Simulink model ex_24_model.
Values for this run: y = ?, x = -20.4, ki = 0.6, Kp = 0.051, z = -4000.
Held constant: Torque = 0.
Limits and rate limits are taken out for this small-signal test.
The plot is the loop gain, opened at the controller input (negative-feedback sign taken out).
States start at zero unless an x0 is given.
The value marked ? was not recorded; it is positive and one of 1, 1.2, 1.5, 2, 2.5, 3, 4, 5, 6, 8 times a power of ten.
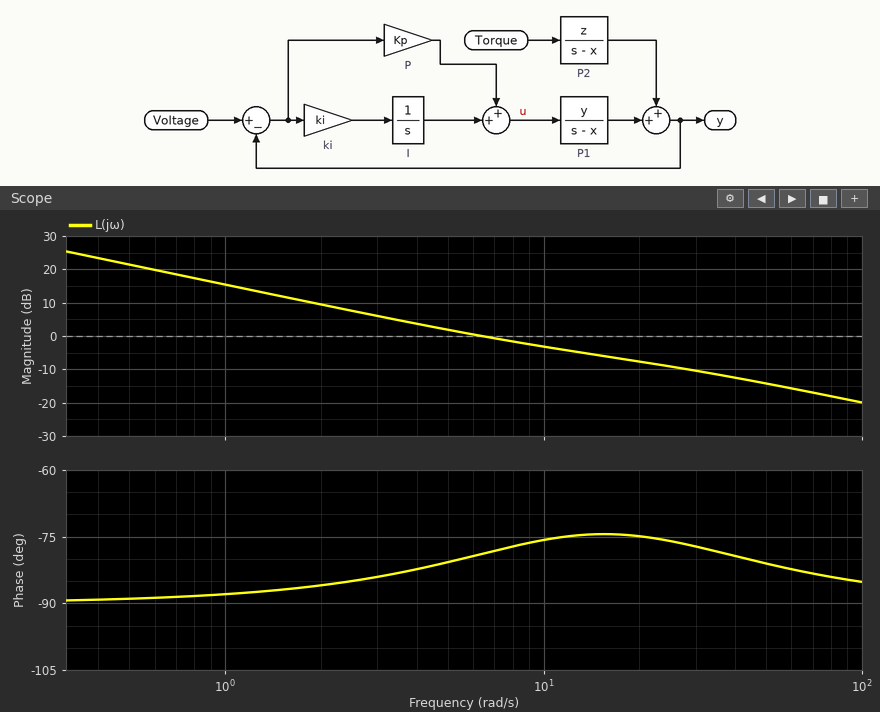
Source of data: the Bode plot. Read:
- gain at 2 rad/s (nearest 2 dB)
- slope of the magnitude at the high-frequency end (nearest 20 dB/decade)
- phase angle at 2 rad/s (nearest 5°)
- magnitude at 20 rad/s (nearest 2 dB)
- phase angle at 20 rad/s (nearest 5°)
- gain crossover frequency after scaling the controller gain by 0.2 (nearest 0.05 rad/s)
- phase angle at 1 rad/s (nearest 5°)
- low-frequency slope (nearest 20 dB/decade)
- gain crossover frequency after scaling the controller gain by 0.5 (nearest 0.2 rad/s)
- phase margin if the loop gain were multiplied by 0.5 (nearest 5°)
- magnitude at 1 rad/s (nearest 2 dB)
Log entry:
10 dB
-20 dB/decade
-85°
-8 dB
-75°
1.20 rad/s
-90°
-20 dB/decade
3.0 rad/s
95°
16 dB
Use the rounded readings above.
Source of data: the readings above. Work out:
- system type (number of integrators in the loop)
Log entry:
1
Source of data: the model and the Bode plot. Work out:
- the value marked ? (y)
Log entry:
200
